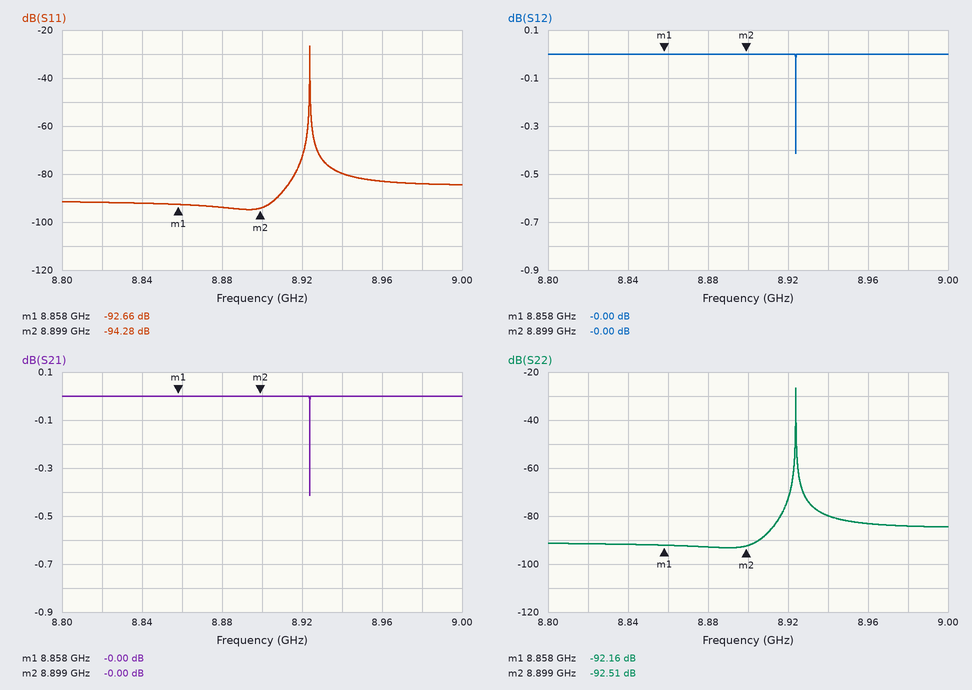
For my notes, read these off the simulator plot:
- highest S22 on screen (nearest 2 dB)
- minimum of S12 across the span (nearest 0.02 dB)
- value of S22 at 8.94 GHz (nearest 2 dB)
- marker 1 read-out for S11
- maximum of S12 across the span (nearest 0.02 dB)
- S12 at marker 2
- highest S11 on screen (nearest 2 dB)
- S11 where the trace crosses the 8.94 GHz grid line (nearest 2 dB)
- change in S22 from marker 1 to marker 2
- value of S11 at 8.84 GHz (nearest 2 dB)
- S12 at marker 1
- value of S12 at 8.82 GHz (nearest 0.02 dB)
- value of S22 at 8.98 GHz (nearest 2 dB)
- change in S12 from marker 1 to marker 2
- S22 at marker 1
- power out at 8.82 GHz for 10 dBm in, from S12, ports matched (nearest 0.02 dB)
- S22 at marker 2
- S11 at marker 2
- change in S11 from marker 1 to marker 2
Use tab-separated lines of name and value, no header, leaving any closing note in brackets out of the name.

highest S22 on screen	-26 dB
minimum of S12 across the span	-0.42 dB
value of S22 at 8.94 GHz	-80 dB
marker 1 read-out for S11	-92.66 dB
maximum of S12 across the span	0.00 dB
S12 at marker 2	-0.00 dB
highest S11 on screen	-26 dB
S11 where the trace crosses the 8.94 GHz grid line	-80 dB
change in S22 from marker 1 to marker 2	-0.35 dB
value of S11 at 8.84 GHz	-92 dB
S12 at marker 1	-0.00 dB
value of S12 at 8.82 GHz	0.00 dB
value of S22 at 8.98 GHz	-84 dB
change in S12 from marker 1 to marker 2	0.00 dB
S22 at marker 1	-92.16 dB
power out at 8.82 GHz for 10 dBm in, from S12, ports matched	10.00 dBm
S22 at marker 2	-92.51 dB
S11 at marker 2	-94.28 dB
change in S11 from marker 1 to marker 2	-1.62 dB
